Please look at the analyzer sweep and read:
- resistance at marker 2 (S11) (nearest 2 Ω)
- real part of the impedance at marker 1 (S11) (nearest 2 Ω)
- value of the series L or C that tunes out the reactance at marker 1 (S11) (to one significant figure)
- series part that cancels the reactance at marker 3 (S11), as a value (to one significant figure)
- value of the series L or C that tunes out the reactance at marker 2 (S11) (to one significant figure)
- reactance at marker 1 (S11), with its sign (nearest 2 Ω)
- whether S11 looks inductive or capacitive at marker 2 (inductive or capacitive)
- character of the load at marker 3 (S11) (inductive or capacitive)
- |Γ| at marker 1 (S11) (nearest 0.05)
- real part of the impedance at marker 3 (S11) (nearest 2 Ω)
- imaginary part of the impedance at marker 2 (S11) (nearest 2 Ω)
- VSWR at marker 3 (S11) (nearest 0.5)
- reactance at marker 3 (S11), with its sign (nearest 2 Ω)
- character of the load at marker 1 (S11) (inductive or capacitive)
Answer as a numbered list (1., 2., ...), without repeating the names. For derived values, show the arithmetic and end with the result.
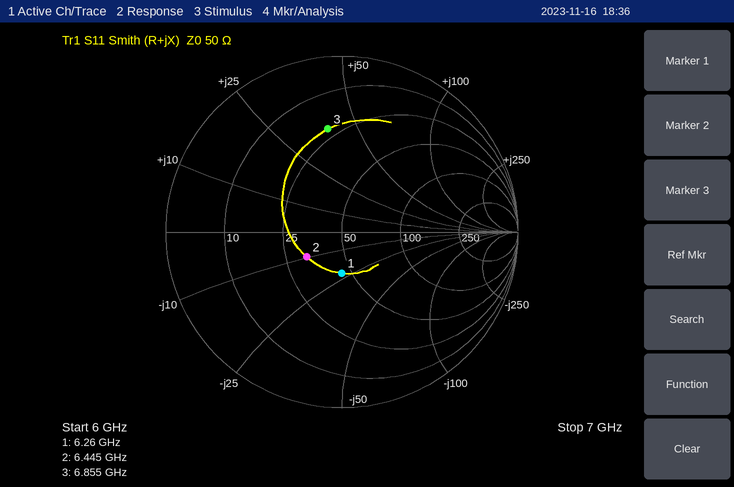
1. 32 Ω
2. 44 Ω
3. L = 22 Ω/(2π × 6.26 GHz) ≈ 559 pH, so 600 pH to one significant figure
4. C = 1/(2π × 6.855 GHz × 38 Ω) ≈ 611 fF, so 600 fF to one significant figure
5. L = 10 Ω/(2π × 6.445 GHz) ≈ 247 pH, so 200 pH to one significant figure
6. -22 Ω
7. capacitive
8. inductive
9. 0.25
10. 22 Ω
11. -10 Ω
12. 4.0
13. +38 Ω
14. capacitive
